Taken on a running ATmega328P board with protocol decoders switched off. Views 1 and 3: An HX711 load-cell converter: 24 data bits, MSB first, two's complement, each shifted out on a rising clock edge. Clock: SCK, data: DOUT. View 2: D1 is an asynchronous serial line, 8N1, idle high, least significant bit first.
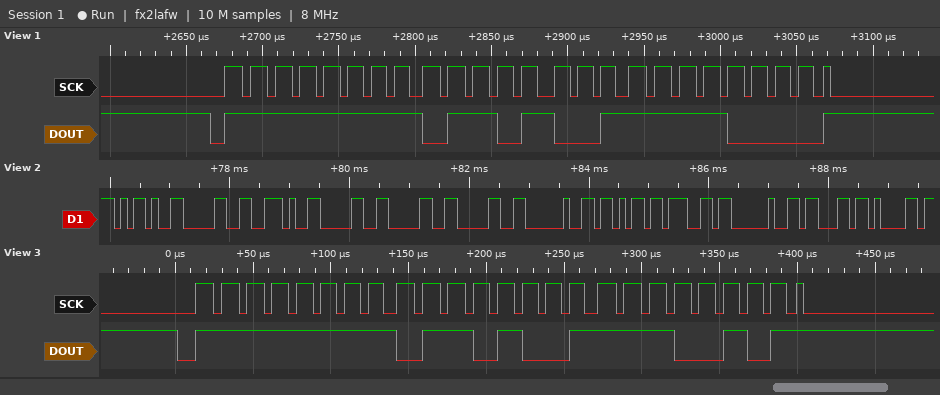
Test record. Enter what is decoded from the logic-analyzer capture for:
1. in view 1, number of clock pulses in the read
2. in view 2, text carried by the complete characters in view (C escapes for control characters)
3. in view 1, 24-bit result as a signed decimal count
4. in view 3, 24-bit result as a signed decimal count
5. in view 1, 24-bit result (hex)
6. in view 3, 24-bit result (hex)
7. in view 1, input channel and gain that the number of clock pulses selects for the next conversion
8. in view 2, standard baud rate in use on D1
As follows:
25
"-0.000 kg ca"
-38416
-38427
0xFF69F0
0xFF69E5
channel A, gain 128
9600 baud
